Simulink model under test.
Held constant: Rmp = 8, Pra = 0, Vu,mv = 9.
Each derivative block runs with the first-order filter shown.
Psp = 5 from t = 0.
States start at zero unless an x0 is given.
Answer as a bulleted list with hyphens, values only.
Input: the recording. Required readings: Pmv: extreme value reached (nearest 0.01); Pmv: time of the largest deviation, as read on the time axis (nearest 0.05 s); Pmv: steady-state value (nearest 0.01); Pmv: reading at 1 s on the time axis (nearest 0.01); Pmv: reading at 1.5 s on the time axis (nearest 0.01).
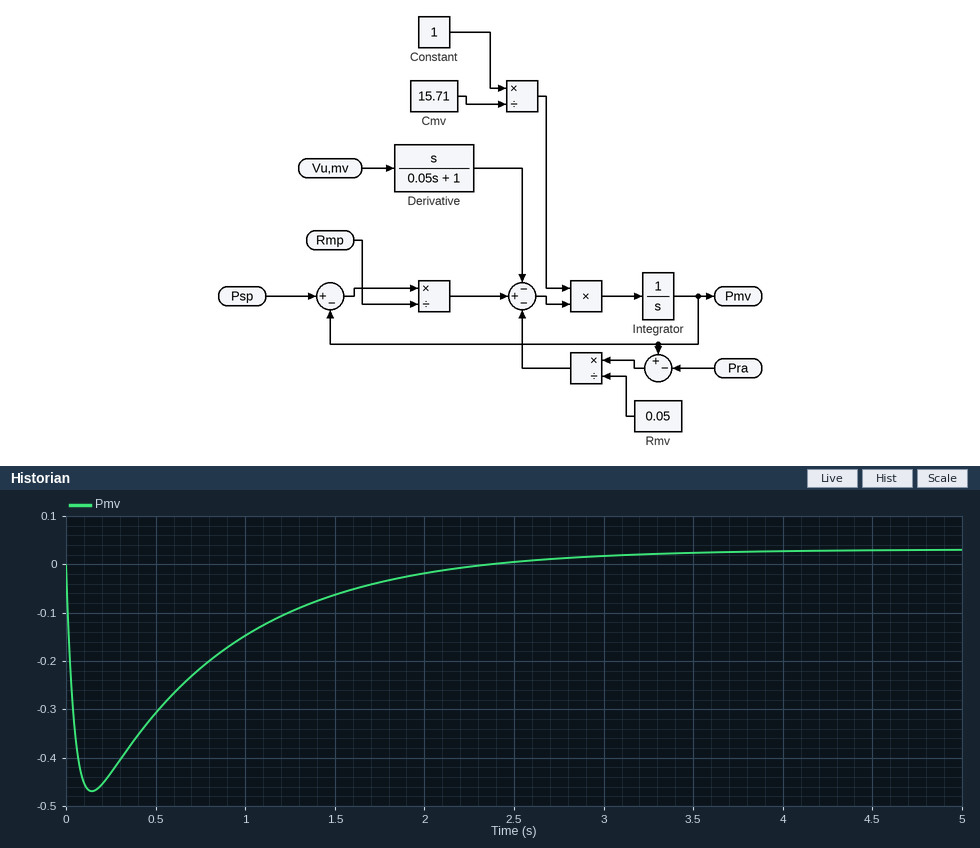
- -0.47
- 0.15 s
- 0.03
- -0.15
- -0.06
